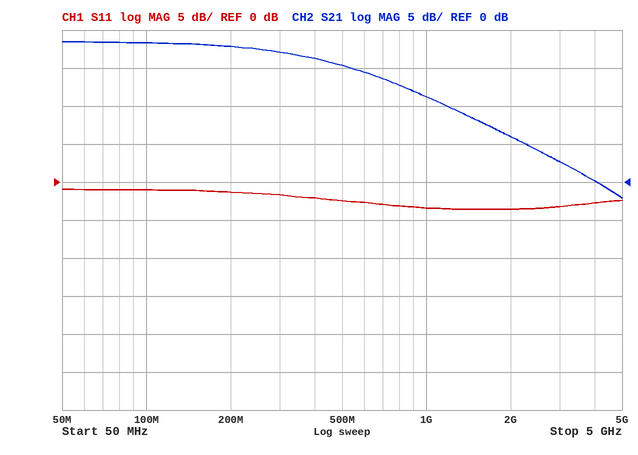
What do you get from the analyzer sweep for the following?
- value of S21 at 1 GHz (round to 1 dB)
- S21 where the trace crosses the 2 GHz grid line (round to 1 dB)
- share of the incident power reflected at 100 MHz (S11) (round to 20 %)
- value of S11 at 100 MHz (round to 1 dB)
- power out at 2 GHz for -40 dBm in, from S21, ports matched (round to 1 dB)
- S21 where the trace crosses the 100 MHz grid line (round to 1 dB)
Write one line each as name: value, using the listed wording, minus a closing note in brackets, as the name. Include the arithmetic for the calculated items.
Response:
value of S21 at 1 GHz: 11 dB
S21 where the trace crosses the 2 GHz grid line: 6 dB
share of the incident power reflected at 100 MHz (S11): 10^(-1/10) ≈ 79.4 %, so 80 % to the nearest 20 %
value of S11 at 100 MHz: -1 dB
power out at 2 GHz for -40 dBm in, from S21, ports matched: -40 dBm + (6 dB) = -34 dBm
S21 where the trace crosses the 100 MHz grid line: 18 dB
